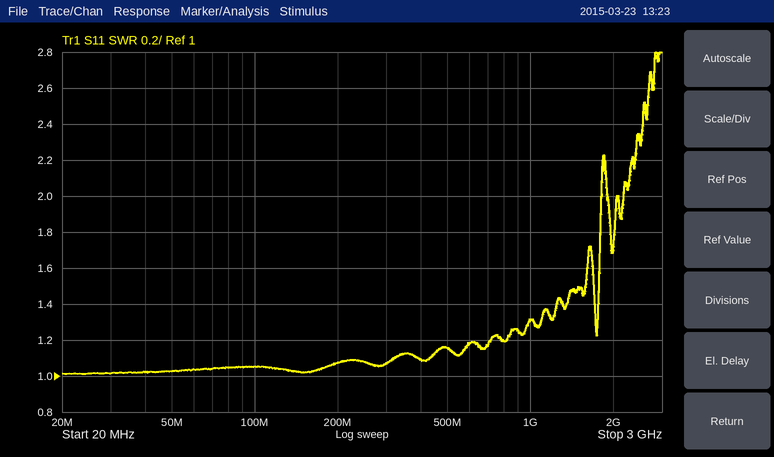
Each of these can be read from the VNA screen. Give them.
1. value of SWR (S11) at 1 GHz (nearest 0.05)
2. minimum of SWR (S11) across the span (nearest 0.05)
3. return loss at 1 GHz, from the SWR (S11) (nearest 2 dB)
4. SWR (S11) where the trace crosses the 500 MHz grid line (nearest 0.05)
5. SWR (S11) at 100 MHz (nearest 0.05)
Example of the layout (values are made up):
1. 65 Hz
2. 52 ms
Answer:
1. 1.30
2. 1.00
3. 18 dB
4. 1.15
5. 1.05
